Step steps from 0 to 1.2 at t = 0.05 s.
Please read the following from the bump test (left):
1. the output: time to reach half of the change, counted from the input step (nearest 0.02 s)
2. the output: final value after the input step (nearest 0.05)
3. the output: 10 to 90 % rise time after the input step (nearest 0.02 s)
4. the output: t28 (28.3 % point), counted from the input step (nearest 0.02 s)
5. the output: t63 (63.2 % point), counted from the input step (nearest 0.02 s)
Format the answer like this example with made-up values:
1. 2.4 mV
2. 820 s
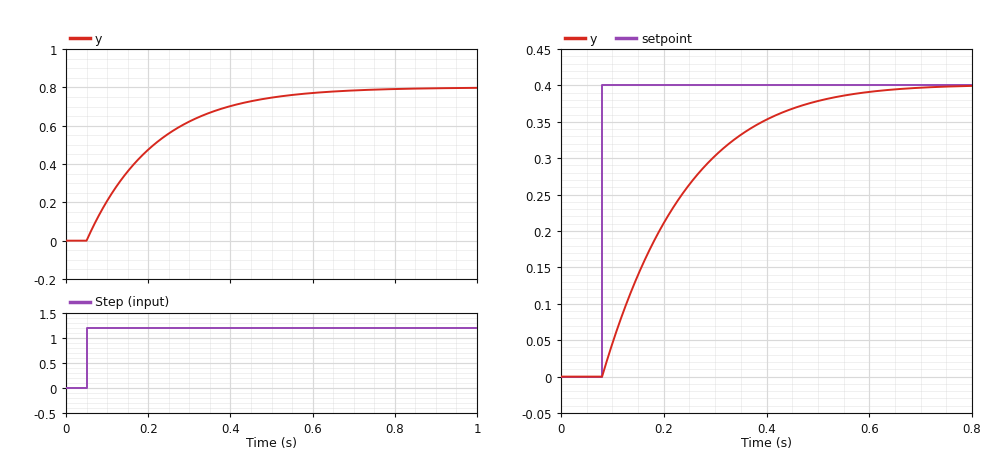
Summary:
1. 0.12 s
2. 0.80
3. 0.36 s
4. 0.06 s
5. 0.16 s
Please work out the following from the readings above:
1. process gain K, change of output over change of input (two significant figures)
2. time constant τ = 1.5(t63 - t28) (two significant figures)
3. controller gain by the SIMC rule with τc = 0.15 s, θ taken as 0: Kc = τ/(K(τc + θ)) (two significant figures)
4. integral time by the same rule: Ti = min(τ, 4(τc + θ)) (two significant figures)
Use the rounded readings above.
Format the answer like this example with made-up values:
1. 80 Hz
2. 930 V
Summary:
1. 0.67
2. 0.15 s
3. 1.5
4. 0.15 s
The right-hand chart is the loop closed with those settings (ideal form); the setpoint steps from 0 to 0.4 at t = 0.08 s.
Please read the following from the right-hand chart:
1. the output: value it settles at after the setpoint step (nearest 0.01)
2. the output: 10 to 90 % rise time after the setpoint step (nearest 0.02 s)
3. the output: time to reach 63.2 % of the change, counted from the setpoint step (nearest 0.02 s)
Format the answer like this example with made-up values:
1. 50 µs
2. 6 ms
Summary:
1. 0.40
2. 0.32 s
3. 0.16 s
